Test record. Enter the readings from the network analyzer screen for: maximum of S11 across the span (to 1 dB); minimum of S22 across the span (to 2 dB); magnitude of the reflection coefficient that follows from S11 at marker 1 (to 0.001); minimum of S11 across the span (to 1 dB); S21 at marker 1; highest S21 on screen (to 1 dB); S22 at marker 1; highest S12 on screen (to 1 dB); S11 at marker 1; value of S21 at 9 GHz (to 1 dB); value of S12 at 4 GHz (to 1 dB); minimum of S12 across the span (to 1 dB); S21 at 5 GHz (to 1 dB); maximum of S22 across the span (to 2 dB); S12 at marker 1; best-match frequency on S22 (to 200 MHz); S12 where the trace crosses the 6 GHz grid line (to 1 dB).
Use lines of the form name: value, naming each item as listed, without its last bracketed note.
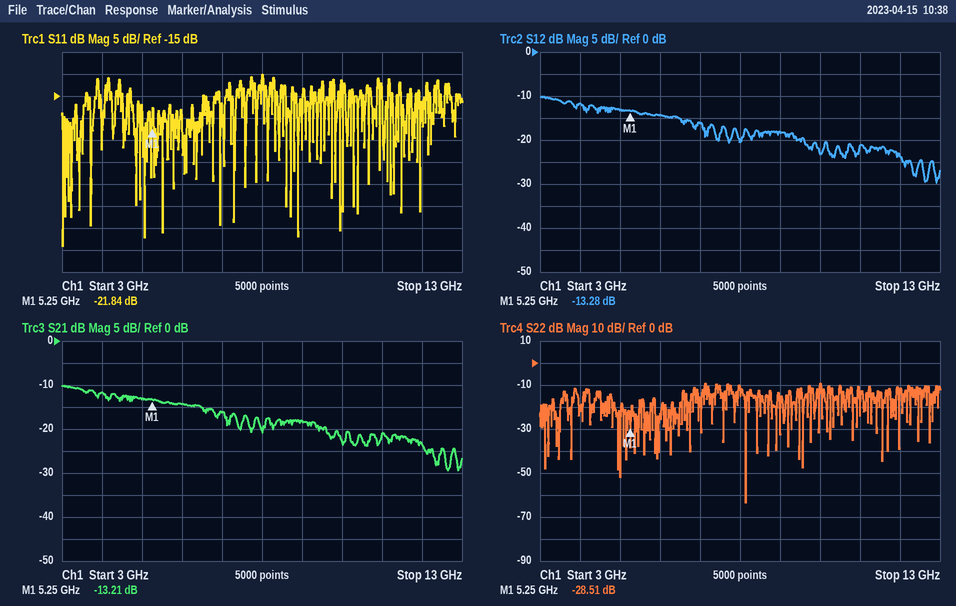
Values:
maximum of S11 across the span: -10 dB
minimum of S22 across the span: -64 dB
magnitude of the reflection coefficient that follows from S11 at marker 1: 0.081
minimum of S11 across the span: -49 dB
S21 at marker 1: -13.21 dB
highest S21 on screen: -10 dB
S22 at marker 1: -28.51 dB
highest S12 on screen: -10 dB
S11 at marker 1: -21.84 dB
value of S21 at 9 GHz: -18 dB
value of S12 at 4 GHz: -12 dB
minimum of S12 across the span: -30 dB
S21 at 5 GHz: -13 dB
maximum of S22 across the span: -10 dB
S12 at marker 1: -13.28 dB
best-match frequency on S22: 8.2 GHz
S12 where the trace crosses the 6 GHz grid line: -14 dB
